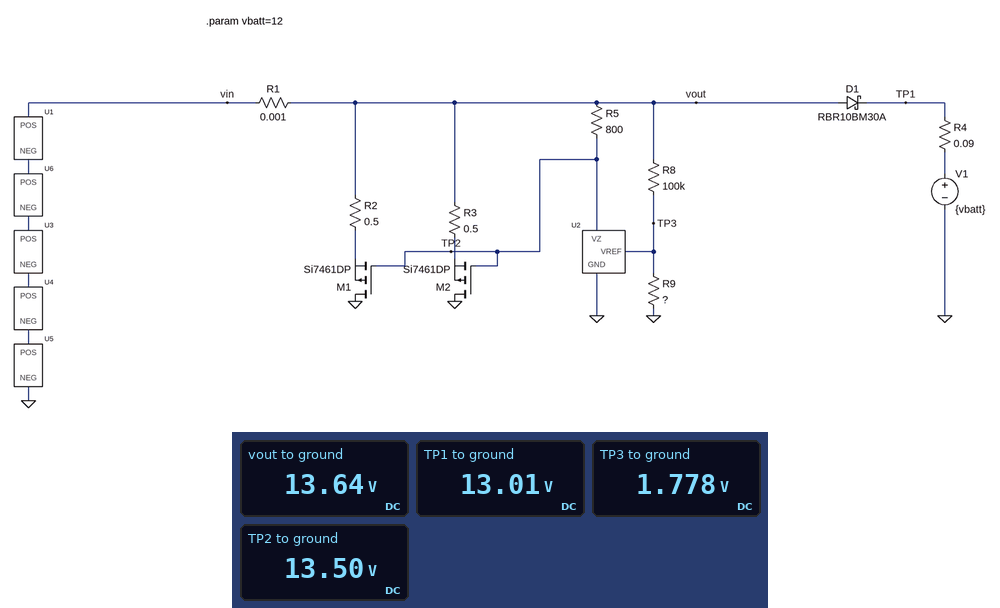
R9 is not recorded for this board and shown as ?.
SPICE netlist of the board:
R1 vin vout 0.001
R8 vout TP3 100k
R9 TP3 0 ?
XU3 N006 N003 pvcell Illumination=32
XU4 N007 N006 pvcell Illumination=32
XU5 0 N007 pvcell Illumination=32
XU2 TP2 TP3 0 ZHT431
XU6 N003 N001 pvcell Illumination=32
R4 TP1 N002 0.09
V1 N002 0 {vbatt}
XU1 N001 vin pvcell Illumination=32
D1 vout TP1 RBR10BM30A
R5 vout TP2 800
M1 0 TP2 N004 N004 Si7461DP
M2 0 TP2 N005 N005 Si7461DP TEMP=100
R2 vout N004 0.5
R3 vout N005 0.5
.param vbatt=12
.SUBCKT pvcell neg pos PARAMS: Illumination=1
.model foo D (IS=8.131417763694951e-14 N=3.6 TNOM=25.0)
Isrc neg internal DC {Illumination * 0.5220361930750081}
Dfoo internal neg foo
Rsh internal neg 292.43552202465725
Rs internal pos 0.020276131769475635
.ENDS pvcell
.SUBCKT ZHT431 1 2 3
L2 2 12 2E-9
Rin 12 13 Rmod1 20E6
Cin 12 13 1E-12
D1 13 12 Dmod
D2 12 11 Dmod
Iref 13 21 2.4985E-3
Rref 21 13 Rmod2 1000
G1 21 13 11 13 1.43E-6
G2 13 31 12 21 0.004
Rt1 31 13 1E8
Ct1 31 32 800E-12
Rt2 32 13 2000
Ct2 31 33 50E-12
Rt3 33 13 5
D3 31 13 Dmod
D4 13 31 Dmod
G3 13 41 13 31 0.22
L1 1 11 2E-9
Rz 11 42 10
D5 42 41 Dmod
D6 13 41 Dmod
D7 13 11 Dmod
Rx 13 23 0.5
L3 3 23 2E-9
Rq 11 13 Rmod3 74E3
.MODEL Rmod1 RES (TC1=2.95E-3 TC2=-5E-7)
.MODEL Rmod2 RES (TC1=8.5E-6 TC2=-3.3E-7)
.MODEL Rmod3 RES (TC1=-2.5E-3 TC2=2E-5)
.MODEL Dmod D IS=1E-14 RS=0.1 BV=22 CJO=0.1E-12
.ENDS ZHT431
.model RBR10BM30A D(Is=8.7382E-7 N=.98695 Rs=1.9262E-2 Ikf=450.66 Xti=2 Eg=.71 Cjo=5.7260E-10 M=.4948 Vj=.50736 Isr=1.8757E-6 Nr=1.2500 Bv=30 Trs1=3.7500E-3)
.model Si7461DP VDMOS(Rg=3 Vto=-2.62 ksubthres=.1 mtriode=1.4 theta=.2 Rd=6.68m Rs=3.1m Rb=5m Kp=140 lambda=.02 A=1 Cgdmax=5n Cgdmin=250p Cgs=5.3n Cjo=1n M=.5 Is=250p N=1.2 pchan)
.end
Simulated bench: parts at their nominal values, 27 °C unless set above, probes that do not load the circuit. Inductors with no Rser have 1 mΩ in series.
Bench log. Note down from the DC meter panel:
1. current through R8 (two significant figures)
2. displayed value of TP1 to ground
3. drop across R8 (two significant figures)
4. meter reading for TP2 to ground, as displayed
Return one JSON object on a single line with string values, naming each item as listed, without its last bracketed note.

{"current through R8": "120 µA", "displayed value of TP1 to ground": "13.01 V", "drop across R8": "12 V", "meter reading for TP2 to ground, as displayed": "13.50 V"}
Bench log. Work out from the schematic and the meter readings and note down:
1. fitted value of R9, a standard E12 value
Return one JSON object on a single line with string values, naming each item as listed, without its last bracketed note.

{"fitted value of R9, a standard E12 value": "15 kΩ"}
